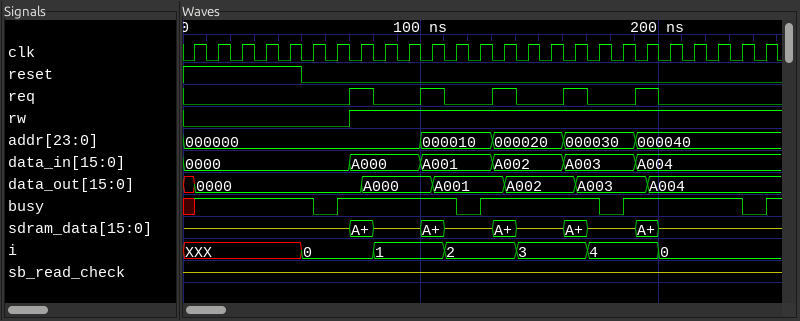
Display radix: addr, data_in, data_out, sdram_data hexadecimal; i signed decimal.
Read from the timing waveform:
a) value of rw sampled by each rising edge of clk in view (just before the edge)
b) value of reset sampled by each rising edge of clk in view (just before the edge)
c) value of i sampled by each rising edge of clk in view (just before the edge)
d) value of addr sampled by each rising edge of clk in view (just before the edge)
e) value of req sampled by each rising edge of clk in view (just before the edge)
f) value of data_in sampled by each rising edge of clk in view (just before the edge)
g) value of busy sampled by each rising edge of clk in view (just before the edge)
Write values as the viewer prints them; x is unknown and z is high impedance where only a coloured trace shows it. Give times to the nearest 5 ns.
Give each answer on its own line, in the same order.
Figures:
0 0 0 0 0 0 0 1 1 1 1 1 1 1 1 1 1 1 1 1 1 1 1 1 1
1 1 1 1 1 0 0 0 0 0 0 0 0 0 0 0 0 0 0 0 0 0 0 0 0
XXX, XXX, XXX, XXX, XXX, 0, 0, 0, 1, 1, 1, 2, 2, 2, 3, 3, 3, 4, 4, 4, 0, 0, 0, 0, 0
000000, 000000, 000000, 000000, 000000, 000000, 000000, 000000, 000000, 000000, 000010, 000010, 000010, 000020, 000020, 000020, 000030, 000030, 000030, 000040, 000040, 000040, 000040, 000040, 000040
0 0 0 0 0 0 0 1 0 0 1 0 0 1 0 0 1 0 0 1 0 0 0 0 0
0000, 0000, 0000, 0000, 0000, 0000, 0000, A000, A000, A000, A001, A001, A001, A002, A002, A002, A003, A003, A003, A004, A004, A004, A004, A004, A004
x 1 1 1 1 1 0 1 1 1 1 1 0 1 1 1 1 1 0 1 1 1 1 1 0
